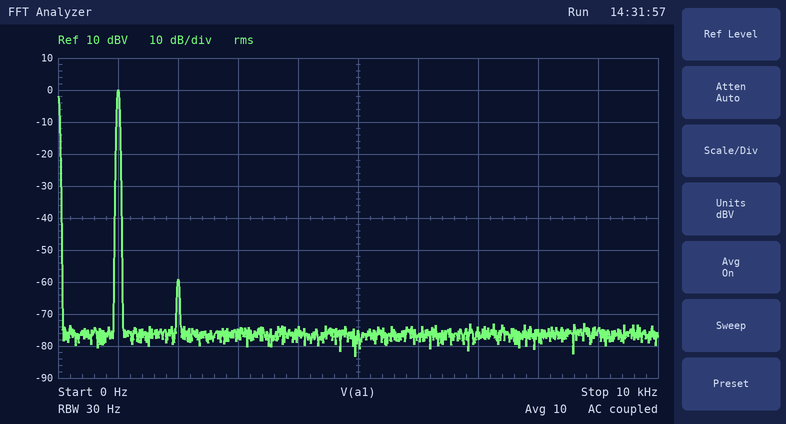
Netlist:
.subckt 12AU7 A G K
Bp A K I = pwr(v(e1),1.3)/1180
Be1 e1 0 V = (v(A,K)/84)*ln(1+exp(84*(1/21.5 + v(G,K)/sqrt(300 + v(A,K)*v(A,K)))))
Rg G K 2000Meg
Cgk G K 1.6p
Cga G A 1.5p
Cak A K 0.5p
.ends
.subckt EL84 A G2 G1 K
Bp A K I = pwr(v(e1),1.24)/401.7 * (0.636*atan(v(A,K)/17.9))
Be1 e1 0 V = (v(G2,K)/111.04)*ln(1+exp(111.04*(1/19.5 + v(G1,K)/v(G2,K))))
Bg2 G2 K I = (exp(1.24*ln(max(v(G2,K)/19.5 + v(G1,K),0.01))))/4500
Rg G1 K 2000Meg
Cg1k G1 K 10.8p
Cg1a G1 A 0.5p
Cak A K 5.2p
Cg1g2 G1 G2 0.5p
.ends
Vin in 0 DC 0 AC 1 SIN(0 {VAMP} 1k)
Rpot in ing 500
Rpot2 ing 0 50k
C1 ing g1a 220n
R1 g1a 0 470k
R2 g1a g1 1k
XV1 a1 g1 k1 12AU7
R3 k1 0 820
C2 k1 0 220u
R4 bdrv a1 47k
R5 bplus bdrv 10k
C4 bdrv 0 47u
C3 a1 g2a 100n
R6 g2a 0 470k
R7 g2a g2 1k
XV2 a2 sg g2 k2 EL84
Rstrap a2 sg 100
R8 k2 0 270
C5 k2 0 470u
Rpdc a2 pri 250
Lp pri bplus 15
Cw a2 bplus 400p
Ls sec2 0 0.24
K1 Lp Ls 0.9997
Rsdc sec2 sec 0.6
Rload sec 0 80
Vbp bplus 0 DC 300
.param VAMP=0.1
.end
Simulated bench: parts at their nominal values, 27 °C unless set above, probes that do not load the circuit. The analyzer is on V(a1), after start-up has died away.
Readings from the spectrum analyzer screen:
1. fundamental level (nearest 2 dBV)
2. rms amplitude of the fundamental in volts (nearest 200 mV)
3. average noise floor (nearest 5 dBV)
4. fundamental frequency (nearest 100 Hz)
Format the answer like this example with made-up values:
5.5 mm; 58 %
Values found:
0 dBV; 1.0 V; -75 dBV; 1.0 kHz
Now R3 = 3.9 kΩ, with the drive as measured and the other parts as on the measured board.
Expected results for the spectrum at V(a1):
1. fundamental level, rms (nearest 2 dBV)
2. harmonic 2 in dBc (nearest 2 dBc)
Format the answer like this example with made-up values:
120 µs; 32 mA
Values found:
-2 dBV; -56 dBc
